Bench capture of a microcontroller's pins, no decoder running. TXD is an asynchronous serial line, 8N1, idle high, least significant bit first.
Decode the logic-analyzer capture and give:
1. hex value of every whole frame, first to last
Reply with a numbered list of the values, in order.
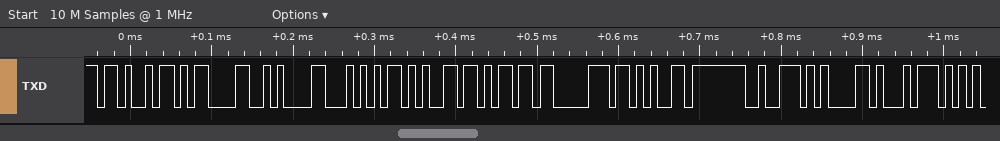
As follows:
1. 0x4B 0x0D 0x0A 0x54 0x65 0x6D 0x70 0x65 0x72 0x61 0x74
